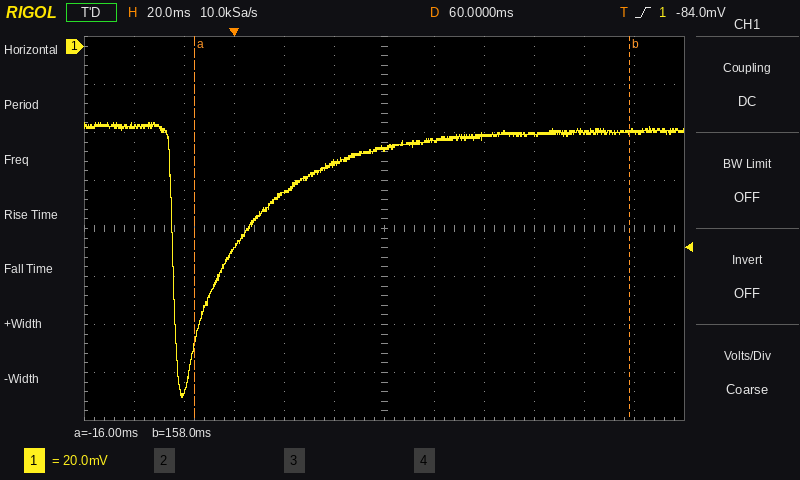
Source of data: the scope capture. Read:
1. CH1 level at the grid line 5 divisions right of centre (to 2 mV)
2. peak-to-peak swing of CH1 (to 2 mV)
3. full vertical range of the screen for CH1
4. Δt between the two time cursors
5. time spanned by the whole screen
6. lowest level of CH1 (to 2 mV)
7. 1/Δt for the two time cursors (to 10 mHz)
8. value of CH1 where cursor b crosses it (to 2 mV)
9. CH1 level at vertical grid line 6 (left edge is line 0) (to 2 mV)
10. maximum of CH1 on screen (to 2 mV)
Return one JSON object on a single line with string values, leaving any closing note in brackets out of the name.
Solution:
{"CH1 level at the grid line 5 divisions right of centre": "-36 mV", "peak-to-peak swing of CH1": "114 mV", "full vertical range of the screen for CH1": "160 mV", "Δt between the two time cursors": "174 ms", "time spanned by the whole screen": "240 ms", "lowest level of CH1": "-146 mV", "1/Δt for the two time cursors": "5.75 Hz", "value of CH1 where cursor b crosses it": "-36 mV", "CH1 level at vertical grid line 6 (left edge is line 0)": "-42 mV", "maximum of CH1 on screen": "-32 mV"}
